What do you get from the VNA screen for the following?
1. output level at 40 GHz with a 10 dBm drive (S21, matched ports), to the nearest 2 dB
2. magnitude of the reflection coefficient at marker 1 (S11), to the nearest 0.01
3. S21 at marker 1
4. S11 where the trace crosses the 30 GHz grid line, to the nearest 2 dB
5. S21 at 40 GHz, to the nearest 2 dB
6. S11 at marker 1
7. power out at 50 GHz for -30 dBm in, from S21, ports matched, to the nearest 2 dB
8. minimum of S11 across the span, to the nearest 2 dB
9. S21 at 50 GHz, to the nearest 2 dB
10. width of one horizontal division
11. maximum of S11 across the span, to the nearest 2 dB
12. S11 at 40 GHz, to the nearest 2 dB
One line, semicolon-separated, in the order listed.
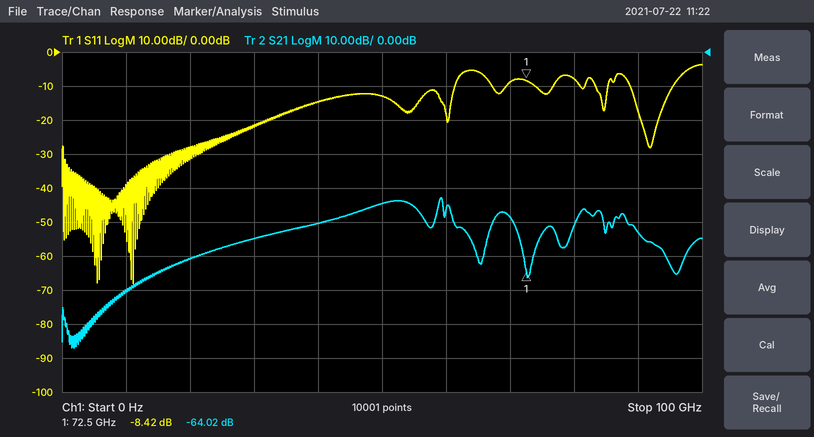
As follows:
-40 dBm; 0.38; -64.02 dB; -22 dB; -50 dB; -8.42 dB; -74 dBm; -68 dB; -44 dB; 10 GHz; -4 dB; -14 dB
